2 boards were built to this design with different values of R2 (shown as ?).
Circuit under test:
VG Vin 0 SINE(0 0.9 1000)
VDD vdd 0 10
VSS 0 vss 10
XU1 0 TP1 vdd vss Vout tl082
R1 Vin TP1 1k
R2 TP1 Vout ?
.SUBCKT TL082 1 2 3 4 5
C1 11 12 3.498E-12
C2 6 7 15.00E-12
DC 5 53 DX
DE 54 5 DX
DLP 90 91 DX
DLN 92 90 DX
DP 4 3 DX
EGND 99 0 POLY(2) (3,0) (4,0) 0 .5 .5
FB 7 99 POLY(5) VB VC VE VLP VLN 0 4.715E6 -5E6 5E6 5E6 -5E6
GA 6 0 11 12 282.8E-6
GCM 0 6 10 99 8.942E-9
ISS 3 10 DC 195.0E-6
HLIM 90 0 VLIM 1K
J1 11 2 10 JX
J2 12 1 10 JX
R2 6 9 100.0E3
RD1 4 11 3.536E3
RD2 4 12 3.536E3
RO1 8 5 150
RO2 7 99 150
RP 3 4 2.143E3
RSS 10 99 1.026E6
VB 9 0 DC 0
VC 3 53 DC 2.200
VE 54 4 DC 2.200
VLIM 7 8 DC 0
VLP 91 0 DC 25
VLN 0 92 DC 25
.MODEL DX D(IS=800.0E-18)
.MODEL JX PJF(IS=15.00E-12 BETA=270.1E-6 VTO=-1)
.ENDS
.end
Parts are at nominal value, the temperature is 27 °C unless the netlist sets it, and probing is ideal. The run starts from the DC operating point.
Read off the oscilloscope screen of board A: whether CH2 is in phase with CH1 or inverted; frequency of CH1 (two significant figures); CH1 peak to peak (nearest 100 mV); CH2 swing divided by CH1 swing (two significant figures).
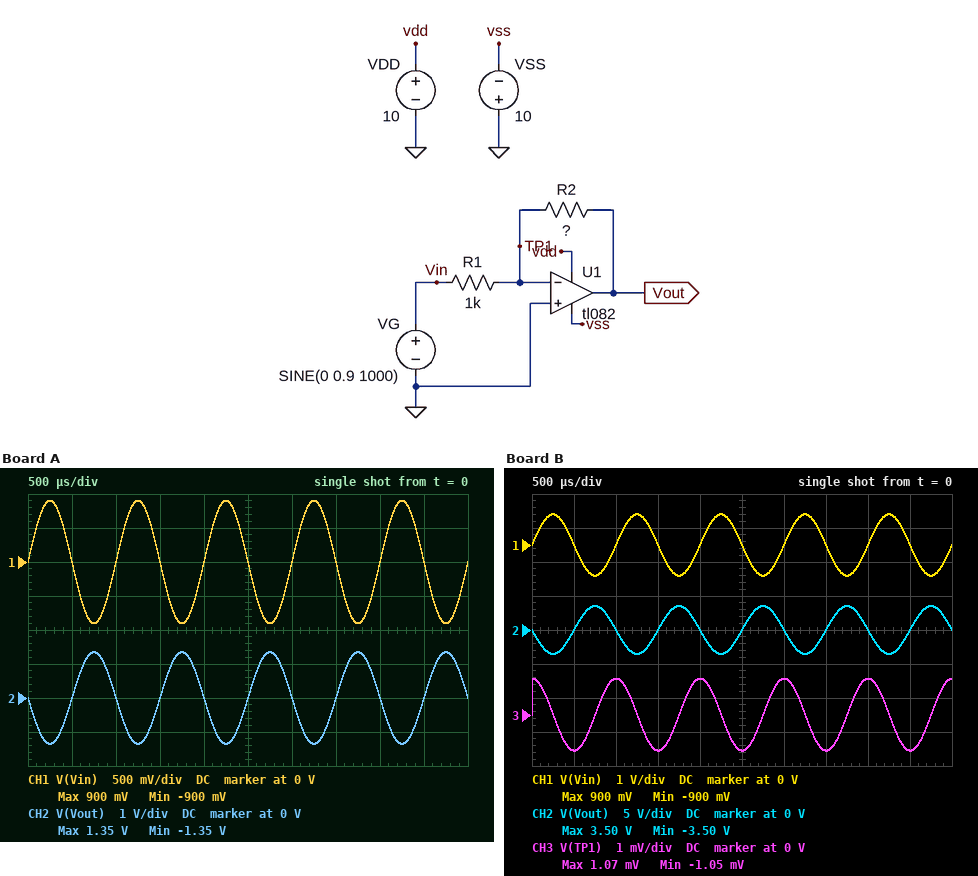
inverted
1.0 kHz
1.8 V
1.5
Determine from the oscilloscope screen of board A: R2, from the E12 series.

1.5 kΩ
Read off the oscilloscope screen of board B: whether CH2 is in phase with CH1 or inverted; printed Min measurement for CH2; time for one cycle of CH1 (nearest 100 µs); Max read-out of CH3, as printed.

inverted
-3.50 V
1.0 ms
1.07 mV
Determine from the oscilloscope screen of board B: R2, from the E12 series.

3.9 kΩ
